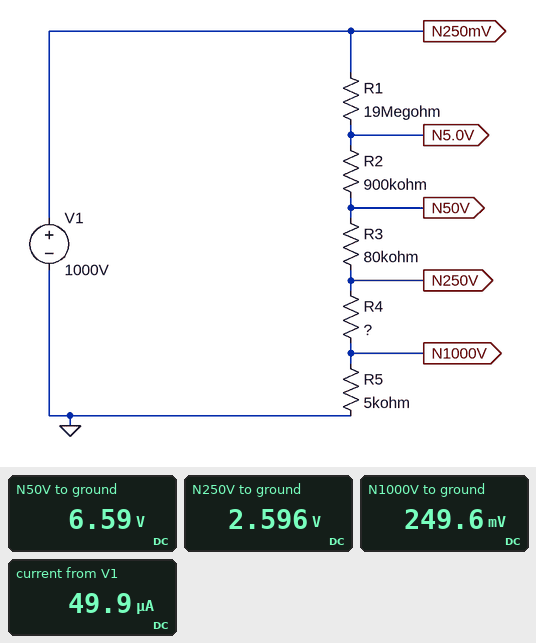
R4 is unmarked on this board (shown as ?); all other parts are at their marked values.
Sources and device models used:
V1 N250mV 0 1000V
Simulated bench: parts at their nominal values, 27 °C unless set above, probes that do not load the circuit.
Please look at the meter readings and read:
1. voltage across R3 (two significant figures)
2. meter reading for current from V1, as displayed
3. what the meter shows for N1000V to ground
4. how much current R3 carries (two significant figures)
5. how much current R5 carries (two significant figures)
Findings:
4.0 V
49.9 µA
249.6 mV
50 µA
50 µA
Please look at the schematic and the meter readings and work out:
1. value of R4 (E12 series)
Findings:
47 kΩ
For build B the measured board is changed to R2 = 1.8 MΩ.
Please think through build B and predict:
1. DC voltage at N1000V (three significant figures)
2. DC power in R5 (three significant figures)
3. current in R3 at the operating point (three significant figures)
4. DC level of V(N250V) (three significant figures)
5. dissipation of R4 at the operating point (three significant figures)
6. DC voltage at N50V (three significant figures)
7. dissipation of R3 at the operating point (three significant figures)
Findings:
239 mV
11.4 µW
47.8 µA
2.48 V
107 µW
6.31 V
183 µW
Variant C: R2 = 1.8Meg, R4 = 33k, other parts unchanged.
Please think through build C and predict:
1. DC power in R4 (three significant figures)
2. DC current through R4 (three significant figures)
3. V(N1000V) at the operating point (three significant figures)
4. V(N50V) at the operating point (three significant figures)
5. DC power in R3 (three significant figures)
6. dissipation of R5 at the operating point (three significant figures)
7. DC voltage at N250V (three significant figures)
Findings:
75.4 µW
47.8 µA
239 mV
5.64 V
183 µW
11.4 µW
1.82 V
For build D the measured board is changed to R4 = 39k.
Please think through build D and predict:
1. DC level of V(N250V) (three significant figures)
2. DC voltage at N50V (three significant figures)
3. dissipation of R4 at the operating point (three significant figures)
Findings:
2.20 V
6.19 V
97.3 µW
